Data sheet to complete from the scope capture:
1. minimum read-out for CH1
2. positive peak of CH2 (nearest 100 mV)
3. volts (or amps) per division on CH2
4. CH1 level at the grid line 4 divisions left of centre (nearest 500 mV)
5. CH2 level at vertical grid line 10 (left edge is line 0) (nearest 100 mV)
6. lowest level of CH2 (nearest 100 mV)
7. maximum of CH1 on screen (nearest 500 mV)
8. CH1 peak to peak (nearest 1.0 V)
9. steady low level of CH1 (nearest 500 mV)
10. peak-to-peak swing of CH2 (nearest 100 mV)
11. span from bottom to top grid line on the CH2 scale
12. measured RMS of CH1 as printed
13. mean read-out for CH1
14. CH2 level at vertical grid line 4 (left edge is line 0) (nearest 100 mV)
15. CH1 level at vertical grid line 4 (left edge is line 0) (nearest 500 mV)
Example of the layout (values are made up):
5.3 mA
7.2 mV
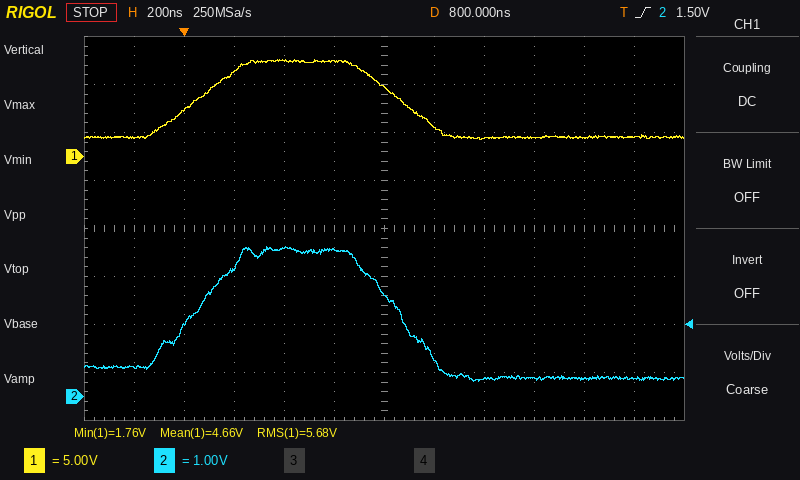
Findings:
1.76 V
3.1 V
1 V
5.0 V
400 mV
300 mV
10.0 V
8.0 V
2.0 V
2.8 V
8 V
5.68 V
4.66 V
3.1 V
10.0 V
